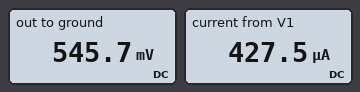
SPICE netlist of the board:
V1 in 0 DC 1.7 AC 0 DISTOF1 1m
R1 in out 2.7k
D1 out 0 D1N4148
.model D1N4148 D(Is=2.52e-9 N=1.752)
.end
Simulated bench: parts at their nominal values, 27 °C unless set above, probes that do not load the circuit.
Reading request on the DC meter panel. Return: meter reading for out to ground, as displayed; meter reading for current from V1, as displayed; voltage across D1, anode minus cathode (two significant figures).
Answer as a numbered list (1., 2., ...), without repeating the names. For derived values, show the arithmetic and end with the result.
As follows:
1. 545.7 mV
2. 427.5 µA
3. 545.7 mV = 550 mV
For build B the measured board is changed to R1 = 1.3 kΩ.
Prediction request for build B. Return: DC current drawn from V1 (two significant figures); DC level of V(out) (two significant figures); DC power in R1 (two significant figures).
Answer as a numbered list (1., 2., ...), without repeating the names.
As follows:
1. 860 µA
2. 580 mV
3. 970 µW
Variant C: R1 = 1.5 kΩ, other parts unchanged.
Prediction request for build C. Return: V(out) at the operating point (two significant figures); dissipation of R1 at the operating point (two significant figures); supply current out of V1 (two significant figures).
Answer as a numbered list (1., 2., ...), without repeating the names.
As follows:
1. 570 mV
2. 850 µW
3. 750 µA
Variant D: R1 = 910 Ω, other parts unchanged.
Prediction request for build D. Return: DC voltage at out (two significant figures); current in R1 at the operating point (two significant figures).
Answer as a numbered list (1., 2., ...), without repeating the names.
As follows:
1. 590 mV
2. 1.2 mA
